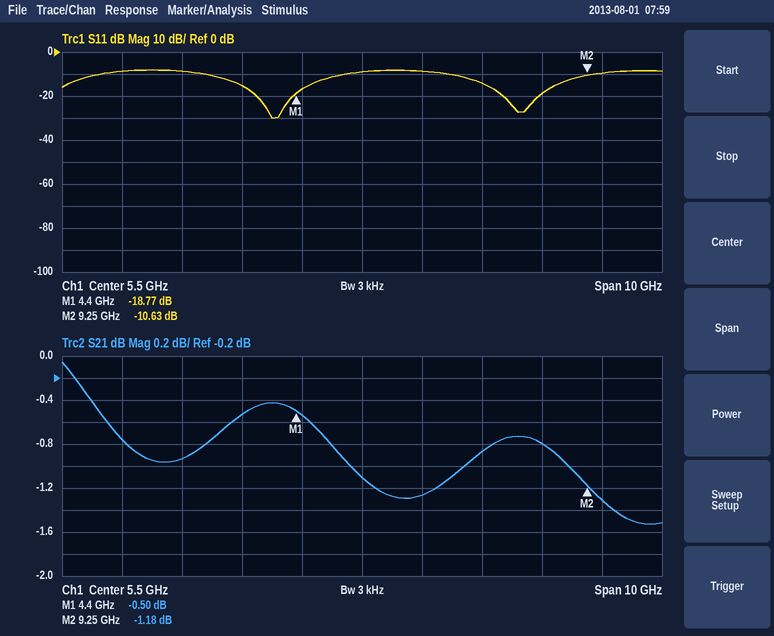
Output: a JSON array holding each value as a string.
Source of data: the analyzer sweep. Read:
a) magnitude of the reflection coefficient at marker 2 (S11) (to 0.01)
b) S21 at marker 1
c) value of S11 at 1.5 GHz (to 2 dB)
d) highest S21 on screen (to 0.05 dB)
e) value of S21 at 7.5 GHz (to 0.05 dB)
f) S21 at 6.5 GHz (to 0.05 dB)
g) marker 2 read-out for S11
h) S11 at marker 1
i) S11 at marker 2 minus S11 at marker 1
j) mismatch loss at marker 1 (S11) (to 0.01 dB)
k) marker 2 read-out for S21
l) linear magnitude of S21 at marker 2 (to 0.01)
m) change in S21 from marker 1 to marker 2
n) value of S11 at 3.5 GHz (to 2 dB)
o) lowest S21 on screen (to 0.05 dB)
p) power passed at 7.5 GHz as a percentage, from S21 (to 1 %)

["0.29", "-0.50 dB", "-8 dB", "-0.05 dB", "-0.85 dB", "-1.25 dB", "-10.63 dB", "-18.77 dB", "8.14 dB", "0.06 dB", "-1.18 dB", "0.87", "-0.68 dB", "-16 dB", "-1.55 dB", "82 %"]
